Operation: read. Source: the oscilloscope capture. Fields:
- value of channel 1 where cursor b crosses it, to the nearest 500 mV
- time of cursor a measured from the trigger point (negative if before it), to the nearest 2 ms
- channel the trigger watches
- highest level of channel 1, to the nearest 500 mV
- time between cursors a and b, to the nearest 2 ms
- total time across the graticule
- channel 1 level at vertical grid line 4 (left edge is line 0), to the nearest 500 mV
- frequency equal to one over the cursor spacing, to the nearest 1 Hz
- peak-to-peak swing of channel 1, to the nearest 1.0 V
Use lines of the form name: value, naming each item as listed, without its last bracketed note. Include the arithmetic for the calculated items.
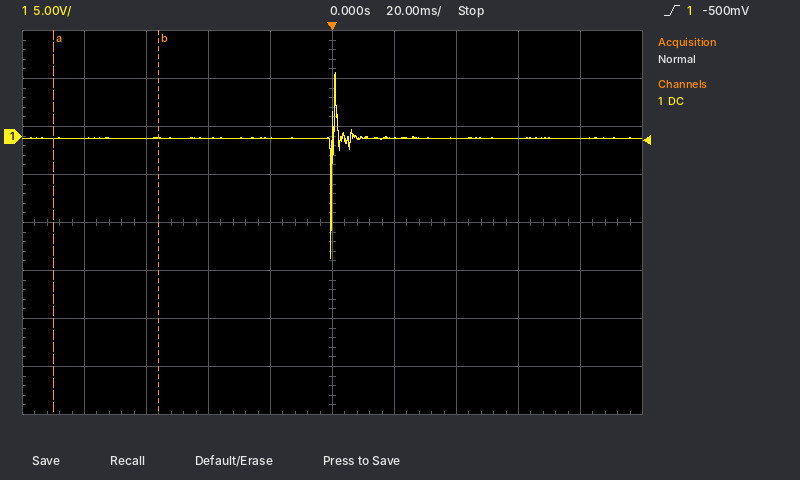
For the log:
value of channel 1 where cursor b crosses it, to the nearest 500 mV: 0.0 V
time of cursor a measured from the trigger point (negative if before it), to the nearest 2 ms: -90 ms
channel the trigger watches: channel 1
highest level of channel 1, to the nearest 500 mV: 6.5 V
time between cursors a and b, to the nearest 2 ms: 34 ms
total time across the graticule: 200 ms
channel 1 level at vertical grid line 4 (left edge is line 0), to the nearest 500 mV: 0.0 V
frequency equal to one over the cursor spacing, to the nearest 1 Hz: 1 / 34 ms ≈ 29 Hz
peak-to-peak swing of channel 1, to the nearest 1.0 V: 19.0 V
